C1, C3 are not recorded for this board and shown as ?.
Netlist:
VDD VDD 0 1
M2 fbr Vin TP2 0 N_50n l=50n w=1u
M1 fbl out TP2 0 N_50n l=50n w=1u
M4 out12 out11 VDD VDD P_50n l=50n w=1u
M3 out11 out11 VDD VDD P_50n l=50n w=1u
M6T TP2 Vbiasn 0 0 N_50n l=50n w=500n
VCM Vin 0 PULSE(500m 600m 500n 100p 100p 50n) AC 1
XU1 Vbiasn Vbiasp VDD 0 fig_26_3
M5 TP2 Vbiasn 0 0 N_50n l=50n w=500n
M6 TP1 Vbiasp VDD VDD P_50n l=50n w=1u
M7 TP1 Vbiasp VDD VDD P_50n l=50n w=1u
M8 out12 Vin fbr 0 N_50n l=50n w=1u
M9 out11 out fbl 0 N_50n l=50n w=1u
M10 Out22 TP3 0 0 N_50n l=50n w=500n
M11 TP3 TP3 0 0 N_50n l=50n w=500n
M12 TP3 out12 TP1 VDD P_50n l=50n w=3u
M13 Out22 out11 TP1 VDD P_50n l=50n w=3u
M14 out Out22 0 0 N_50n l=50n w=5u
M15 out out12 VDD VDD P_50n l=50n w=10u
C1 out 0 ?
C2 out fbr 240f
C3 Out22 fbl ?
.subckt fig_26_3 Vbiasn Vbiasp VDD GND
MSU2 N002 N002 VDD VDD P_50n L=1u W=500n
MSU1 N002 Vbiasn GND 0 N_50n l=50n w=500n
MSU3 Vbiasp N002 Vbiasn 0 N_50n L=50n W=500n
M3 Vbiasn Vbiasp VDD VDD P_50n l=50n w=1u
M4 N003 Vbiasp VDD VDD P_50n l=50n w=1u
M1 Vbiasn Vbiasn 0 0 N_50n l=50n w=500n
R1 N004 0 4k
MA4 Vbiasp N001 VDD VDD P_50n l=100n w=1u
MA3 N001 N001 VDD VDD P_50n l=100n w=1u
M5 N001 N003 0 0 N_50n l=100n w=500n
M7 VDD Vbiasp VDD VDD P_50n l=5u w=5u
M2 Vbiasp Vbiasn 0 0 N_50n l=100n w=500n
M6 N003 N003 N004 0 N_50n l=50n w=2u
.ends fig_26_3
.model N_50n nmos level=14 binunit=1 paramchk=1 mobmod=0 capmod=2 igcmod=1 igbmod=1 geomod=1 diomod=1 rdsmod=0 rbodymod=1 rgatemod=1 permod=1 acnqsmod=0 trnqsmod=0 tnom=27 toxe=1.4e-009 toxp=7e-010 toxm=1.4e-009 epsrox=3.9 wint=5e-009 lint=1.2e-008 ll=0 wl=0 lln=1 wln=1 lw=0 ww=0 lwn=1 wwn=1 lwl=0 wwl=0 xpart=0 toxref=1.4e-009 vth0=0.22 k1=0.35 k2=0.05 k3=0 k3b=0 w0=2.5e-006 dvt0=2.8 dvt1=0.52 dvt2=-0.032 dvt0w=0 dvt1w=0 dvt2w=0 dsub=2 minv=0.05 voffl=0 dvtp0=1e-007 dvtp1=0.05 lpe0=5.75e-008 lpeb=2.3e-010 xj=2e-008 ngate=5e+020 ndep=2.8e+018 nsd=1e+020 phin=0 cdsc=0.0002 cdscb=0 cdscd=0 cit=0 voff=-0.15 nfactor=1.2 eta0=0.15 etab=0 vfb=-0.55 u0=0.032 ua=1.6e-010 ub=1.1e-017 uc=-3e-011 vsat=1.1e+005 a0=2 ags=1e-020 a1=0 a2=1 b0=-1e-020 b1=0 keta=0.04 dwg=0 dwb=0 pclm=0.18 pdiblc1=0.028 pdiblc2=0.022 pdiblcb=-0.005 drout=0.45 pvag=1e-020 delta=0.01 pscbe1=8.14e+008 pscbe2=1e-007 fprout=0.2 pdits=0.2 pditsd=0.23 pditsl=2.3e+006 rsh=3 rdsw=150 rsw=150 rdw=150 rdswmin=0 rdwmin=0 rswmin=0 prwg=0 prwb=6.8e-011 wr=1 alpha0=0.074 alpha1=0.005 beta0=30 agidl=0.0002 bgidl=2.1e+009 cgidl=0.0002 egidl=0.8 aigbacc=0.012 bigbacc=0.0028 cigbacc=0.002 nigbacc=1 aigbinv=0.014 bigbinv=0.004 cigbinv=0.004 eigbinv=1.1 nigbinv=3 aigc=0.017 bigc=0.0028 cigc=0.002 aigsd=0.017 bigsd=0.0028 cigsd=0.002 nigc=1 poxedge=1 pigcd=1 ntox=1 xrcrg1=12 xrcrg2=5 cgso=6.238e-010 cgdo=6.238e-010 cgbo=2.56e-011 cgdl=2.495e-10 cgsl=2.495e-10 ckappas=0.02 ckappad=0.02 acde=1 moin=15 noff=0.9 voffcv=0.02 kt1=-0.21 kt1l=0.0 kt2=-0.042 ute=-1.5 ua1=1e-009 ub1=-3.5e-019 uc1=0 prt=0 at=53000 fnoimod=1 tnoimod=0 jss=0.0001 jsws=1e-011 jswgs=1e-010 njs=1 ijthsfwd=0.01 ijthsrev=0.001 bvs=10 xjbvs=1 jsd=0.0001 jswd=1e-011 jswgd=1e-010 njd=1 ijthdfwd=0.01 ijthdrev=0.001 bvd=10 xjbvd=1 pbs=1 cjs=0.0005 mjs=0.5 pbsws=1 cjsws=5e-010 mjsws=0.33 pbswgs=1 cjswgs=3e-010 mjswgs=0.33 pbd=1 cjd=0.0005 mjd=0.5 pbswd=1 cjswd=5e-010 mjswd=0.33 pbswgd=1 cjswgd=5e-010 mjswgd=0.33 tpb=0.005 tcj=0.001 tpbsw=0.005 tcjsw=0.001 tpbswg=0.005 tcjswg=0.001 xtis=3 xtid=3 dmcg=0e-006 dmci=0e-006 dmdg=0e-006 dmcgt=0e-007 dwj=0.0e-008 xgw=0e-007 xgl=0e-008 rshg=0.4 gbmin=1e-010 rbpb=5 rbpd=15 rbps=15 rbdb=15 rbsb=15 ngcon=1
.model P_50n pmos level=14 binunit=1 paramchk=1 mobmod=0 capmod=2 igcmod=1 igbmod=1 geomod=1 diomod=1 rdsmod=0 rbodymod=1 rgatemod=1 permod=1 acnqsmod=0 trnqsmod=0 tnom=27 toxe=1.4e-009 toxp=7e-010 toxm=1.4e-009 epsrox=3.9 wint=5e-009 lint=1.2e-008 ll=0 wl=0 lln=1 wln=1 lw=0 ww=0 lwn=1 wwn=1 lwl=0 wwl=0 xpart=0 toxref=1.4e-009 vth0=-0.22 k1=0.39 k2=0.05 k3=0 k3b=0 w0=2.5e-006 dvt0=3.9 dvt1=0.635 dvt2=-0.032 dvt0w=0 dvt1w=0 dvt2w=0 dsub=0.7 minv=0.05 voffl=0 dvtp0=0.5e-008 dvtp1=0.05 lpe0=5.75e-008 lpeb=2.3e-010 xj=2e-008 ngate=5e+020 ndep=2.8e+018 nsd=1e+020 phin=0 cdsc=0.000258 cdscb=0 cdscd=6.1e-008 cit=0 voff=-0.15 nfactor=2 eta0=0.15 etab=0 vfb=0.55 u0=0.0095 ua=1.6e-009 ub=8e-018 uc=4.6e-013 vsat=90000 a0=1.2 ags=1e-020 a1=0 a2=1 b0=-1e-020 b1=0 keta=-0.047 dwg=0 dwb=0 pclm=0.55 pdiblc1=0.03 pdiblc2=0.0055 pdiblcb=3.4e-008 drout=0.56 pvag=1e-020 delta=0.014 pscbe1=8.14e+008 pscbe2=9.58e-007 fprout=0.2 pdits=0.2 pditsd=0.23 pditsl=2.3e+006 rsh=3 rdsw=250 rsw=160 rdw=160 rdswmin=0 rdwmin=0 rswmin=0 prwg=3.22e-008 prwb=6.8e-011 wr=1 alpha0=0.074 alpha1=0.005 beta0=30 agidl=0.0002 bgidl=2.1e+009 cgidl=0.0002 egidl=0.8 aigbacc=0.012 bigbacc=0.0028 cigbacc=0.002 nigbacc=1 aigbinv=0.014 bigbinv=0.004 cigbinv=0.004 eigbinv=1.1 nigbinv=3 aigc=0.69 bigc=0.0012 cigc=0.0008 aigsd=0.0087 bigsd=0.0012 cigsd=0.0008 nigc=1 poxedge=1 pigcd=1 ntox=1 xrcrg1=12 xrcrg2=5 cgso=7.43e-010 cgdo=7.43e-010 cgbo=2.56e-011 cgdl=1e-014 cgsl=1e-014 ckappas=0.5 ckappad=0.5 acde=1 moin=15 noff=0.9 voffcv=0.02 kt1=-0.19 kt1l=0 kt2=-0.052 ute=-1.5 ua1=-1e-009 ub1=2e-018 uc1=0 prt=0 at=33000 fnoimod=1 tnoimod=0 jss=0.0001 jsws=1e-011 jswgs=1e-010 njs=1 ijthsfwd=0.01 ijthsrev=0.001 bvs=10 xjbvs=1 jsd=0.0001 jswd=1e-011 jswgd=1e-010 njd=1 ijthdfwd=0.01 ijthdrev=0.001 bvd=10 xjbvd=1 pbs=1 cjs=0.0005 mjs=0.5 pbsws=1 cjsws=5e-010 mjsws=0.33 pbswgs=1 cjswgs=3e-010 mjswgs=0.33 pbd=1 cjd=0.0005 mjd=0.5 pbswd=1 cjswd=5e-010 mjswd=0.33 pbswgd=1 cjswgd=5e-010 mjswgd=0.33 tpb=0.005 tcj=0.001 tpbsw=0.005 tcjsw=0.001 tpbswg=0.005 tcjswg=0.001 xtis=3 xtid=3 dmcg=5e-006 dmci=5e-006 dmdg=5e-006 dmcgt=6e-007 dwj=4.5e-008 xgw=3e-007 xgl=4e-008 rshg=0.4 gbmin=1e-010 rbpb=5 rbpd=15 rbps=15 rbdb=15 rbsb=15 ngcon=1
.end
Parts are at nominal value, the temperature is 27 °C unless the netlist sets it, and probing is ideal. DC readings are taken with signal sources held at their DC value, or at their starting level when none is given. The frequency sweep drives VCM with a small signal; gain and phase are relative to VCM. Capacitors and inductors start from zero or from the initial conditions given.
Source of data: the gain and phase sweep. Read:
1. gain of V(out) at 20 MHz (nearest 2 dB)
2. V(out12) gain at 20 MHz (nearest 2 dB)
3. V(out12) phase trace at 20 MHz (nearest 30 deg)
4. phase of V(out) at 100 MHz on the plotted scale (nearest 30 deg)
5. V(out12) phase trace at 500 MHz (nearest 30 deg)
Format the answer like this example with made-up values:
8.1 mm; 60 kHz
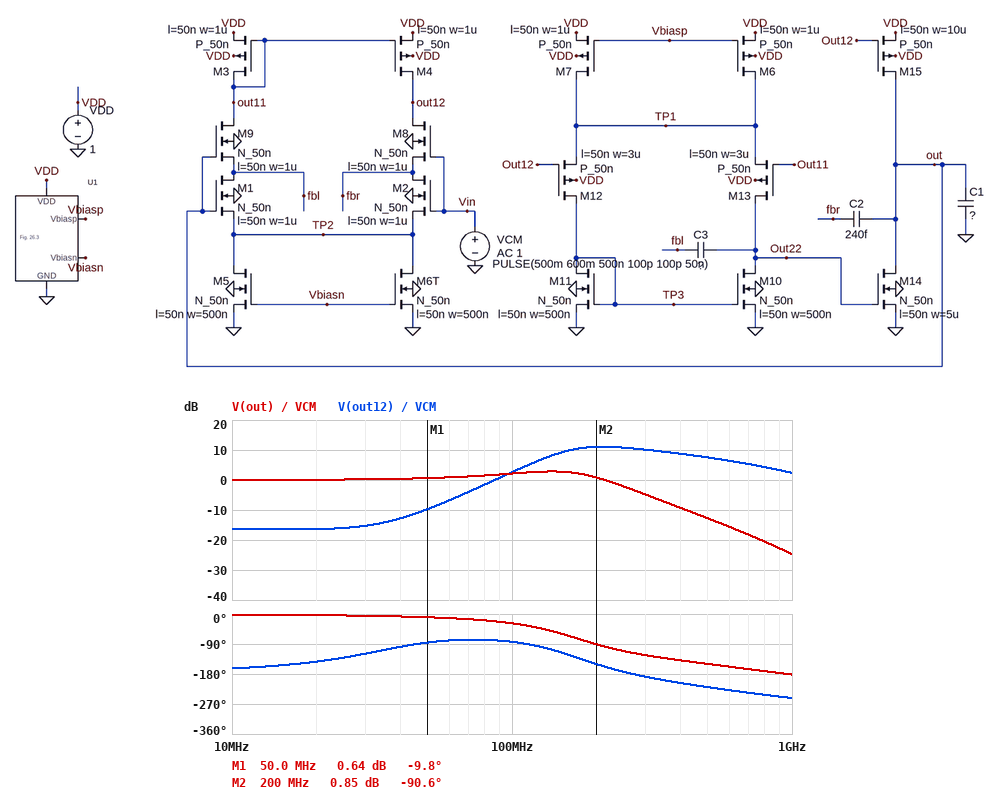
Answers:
0 dB; -16 dB; -150 deg; -30 deg; -210 deg
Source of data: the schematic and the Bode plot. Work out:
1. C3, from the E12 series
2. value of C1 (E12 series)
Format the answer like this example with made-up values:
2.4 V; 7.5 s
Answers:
82 fF; 8.2 pF
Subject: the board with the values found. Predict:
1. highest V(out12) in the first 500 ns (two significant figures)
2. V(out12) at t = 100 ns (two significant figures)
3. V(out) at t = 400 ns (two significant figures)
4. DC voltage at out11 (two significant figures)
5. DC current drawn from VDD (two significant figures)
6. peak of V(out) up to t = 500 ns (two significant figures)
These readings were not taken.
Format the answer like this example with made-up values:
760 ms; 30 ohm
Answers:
1.0 V; 710 mV; 500 mV; 600 mV; 260 µA; 630 mV
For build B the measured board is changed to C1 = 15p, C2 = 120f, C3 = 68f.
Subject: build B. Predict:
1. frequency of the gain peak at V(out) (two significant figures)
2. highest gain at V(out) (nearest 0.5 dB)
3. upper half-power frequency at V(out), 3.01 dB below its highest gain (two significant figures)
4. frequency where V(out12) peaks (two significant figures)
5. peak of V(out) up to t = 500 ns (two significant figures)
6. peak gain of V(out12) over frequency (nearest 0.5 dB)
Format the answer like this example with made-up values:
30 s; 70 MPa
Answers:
120 MHz; 6.5 dB; 150 MHz; 130 MHz; 570 mV; 14.5 dB
